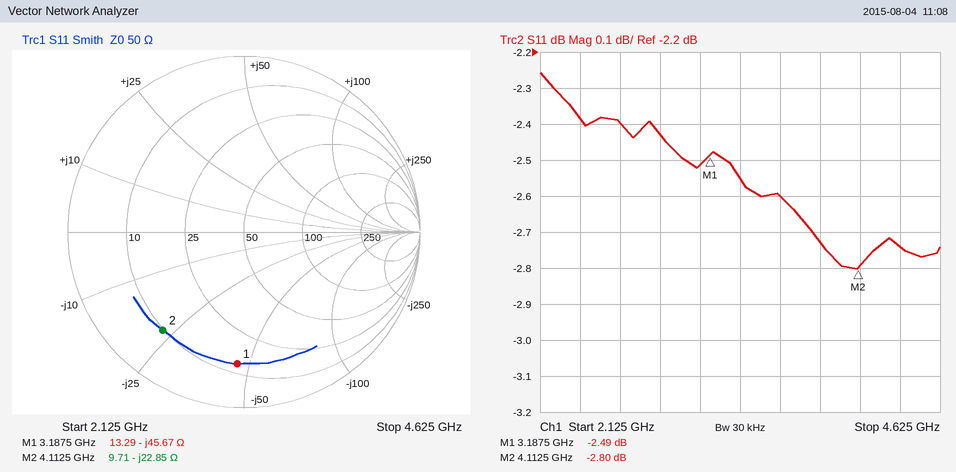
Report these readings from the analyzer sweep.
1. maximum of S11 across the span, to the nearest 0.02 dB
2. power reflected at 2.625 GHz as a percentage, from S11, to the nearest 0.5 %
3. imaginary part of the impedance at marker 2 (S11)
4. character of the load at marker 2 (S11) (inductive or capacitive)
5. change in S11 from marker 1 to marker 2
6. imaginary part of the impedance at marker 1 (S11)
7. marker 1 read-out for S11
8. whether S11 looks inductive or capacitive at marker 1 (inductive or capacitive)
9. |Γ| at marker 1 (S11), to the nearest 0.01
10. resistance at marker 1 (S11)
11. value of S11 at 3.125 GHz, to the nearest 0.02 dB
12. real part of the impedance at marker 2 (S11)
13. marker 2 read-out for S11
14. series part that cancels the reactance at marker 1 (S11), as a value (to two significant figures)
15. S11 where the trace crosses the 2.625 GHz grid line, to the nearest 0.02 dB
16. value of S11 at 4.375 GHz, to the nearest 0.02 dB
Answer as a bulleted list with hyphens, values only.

- -2.26 dB
- 57.5 %
- -22.85 Ω
- capacitive
- -0.31 dB
- -45.67 Ω
- -2.49 dB
- capacitive
- 0.75
- 13.29 Ω
- -2.52 dB
- 9.71 Ω
- -2.80 dB
- 2.3 nH
- -2.40 dB
- -2.74 dB
